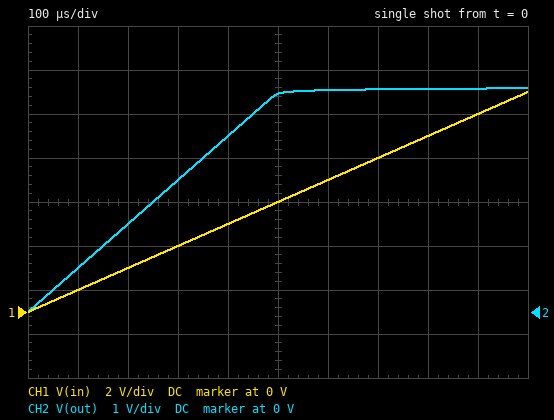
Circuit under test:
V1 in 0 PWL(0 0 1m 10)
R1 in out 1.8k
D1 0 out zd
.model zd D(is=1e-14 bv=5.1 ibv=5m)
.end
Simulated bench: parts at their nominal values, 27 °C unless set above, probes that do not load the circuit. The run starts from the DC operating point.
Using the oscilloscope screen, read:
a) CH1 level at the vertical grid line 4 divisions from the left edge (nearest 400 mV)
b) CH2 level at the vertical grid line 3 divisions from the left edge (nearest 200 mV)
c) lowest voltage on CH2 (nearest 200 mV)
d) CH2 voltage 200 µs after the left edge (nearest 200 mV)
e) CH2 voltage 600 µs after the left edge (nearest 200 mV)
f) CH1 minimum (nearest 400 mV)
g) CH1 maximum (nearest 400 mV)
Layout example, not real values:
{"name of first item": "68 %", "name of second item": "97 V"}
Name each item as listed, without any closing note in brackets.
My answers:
{"CH1 level at the vertical grid line 4 divisions from the left edge": "4.0 V", "CH2 level at the vertical grid line 3 divisions from the left edge": "3.0 V", "lowest voltage on CH2": "0 V", "CH2 voltage 200 µs after the left edge": "2.0 V", "CH2 voltage 600 µs after the left edge": "5.0 V", "CH1 minimum": "0 V", "CH1 maximum": "10.0 V"}
